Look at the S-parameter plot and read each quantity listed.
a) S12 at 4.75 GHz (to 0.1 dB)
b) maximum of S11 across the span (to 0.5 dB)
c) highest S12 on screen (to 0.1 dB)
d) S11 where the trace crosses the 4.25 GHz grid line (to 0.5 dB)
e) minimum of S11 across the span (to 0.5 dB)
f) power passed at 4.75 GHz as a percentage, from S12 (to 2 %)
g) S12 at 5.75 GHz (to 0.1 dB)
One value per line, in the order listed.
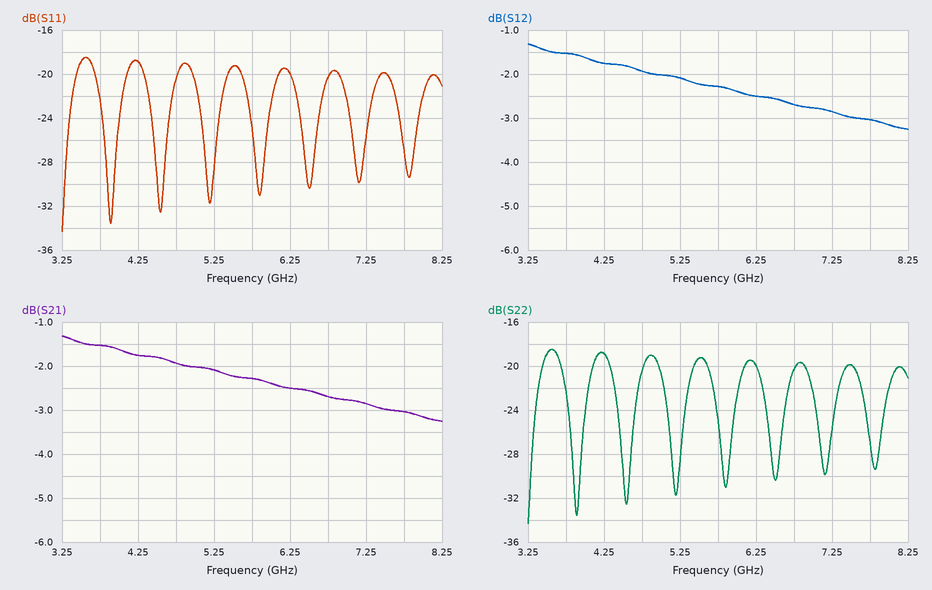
-1.9 dB
-18.5 dB
-1.3 dB
-19.0 dB
-34.5 dB
64 %
-2.3 dB
